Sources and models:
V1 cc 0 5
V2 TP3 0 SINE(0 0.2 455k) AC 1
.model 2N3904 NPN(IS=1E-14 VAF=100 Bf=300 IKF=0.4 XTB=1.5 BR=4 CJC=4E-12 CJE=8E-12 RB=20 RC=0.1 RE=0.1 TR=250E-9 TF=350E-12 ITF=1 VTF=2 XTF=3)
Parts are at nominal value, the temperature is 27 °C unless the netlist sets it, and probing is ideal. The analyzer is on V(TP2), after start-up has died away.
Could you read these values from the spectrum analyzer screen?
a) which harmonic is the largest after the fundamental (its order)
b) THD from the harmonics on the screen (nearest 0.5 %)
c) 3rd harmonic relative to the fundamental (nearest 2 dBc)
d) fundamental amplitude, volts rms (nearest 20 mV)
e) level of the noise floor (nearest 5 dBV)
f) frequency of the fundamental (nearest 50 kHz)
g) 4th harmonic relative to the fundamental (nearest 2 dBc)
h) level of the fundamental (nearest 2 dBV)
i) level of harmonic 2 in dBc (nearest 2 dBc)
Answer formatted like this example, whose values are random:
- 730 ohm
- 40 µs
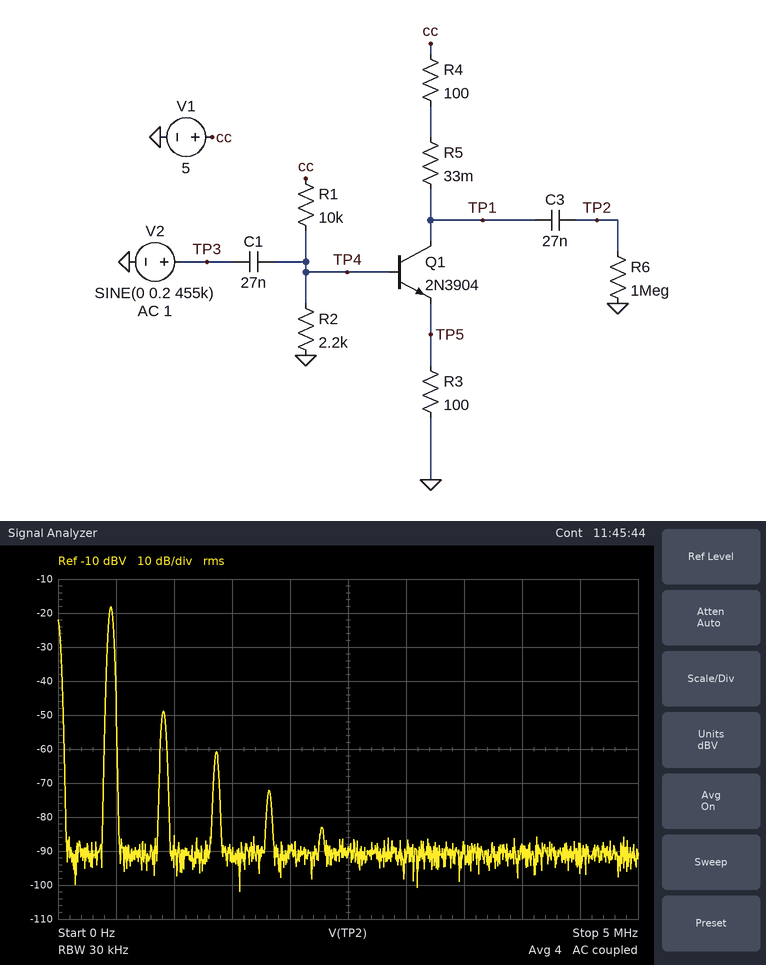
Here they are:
- 2
- 3.0 %
- -42 dBc
- 120 mV
- -90 dBV
- 450 kHz
- -54 dBc
- -18 dBV
- -30 dBc
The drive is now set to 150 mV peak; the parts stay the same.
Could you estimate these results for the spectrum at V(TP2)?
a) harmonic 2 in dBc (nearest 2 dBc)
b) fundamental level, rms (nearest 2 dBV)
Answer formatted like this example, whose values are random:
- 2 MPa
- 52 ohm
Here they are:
- -34 dBc
- -20 dBV
